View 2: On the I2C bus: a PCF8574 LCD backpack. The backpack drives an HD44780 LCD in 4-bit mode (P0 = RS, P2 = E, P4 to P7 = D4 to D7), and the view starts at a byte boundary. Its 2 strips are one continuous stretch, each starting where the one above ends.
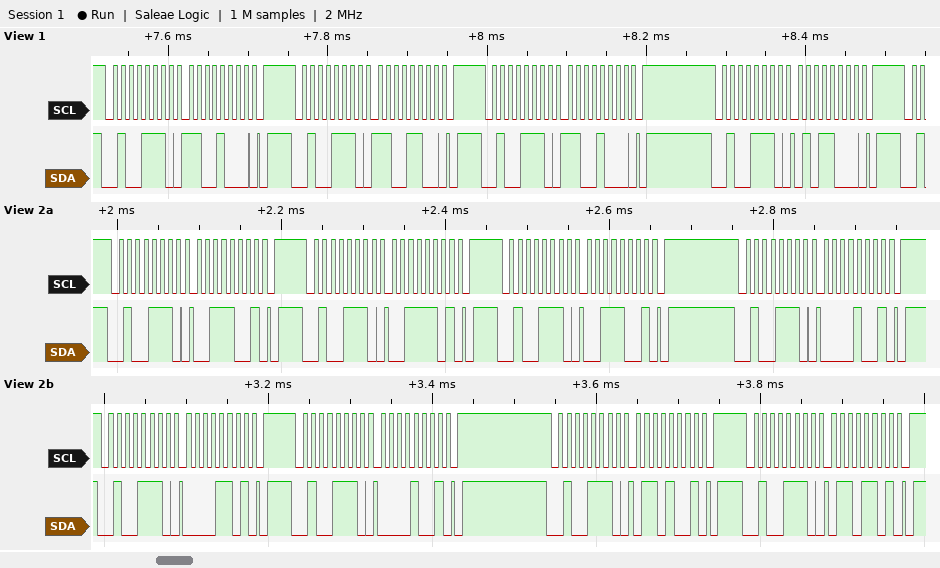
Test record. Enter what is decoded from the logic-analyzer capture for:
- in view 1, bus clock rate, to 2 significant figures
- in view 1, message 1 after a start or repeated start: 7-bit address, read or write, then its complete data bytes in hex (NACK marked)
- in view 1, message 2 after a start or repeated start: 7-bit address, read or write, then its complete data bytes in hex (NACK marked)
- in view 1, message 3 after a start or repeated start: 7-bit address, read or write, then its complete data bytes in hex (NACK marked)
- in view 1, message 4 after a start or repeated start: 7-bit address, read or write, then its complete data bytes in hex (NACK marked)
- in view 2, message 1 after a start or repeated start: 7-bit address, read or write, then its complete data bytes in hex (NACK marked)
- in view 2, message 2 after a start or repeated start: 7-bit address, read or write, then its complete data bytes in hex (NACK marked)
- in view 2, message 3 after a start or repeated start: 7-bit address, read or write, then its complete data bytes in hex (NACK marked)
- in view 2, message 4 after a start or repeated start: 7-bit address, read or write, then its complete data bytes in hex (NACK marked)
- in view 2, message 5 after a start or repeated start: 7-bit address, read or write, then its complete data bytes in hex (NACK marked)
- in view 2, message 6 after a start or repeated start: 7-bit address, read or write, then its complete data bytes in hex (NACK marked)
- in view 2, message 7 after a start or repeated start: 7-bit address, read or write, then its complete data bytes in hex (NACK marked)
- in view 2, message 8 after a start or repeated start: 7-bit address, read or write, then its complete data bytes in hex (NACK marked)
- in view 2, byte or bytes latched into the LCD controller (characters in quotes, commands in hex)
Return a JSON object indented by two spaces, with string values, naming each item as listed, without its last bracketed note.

{
  "in view 1, bus clock rate, to 2 significant figures": "100 kHz",
  "in view 1, message 1 after a start or repeated start: 7-bit address, read or write, then its complete data bytes in hex": "0x27 write: C8",
  "in view 1, message 2 after a start or repeated start: 7-bit address, read or write, then its complete data bytes in hex": "0x27 write: CC",
  "in view 1, message 3 after a start or repeated start: 7-bit address, read or write, then its complete data bytes in hex": "0x27 write: C8",
  "in view 1, message 4 after a start or repeated start: 7-bit address, read or write, then its complete data bytes in hex": "0x27 write: 58",
  "in view 2, message 1 after a start or repeated start: 7-bit address, read or write, then its complete data bytes in hex": "0x27 write: 39",
  "in view 2, message 2 after a start or repeated start: 7-bit address, read or write, then its complete data bytes in hex": "0x27 write: 3D",
  "in view 2, message 3 after a start or repeated start: 7-bit address, read or write, then its complete data bytes in hex": "0x27 write: 39",
  "in view 2, message 4 after a start or repeated start: 7-bit address, read or write, then its complete data bytes in hex": "0x27 write: 09",
  "in view 2, message 5 after a start or repeated start: 7-bit address, read or write, then its complete data bytes in hex": "0x27 write: 0D",
  "in view 2, message 6 after a start or repeated start: 7-bit address, read or write, then its complete data bytes in hex": "0x27 write: 09",
  "in view 2, message 7 after a start or repeated start: 7-bit address, read or write, then its complete data bytes in hex": "0x27 write: 69",
  "in view 2, message 8 after a start or repeated start: 7-bit address, read or write, then its complete data bytes in hex": "0x27 write: 6D",
  "in view 2, byte or bytes latched into the LCD controller": "'0'"
}
